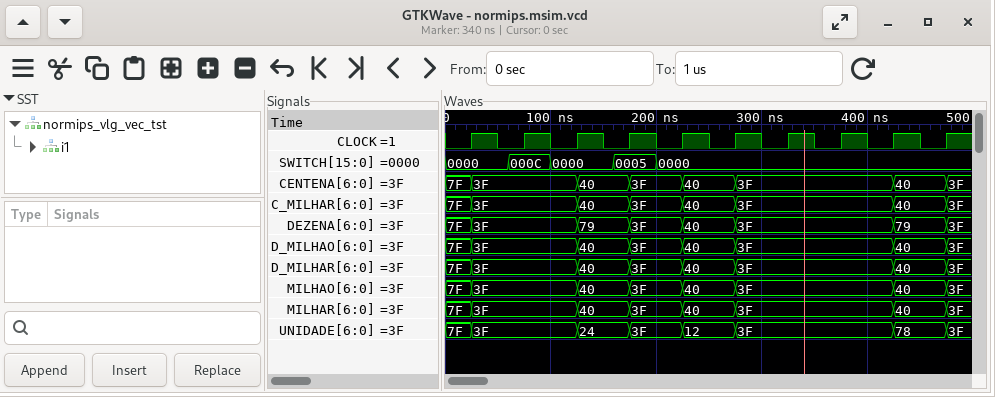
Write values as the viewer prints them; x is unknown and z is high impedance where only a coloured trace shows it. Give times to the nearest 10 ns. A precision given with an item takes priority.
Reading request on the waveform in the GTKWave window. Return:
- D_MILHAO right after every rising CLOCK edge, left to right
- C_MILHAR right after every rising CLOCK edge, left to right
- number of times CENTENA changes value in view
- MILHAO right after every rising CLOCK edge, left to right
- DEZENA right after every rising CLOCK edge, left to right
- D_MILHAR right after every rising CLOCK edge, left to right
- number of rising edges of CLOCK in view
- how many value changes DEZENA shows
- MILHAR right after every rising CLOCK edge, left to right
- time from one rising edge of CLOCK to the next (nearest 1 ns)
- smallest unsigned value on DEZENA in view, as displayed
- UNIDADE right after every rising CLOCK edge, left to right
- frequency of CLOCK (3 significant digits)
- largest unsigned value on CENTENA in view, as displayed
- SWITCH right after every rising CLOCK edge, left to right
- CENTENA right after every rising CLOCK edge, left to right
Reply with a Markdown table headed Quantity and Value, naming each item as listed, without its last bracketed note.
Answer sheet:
| Quantity | Value |
|---|---|
| D_MILHAO right after every rising CLOCK edge, left to right | 3F, 3F, 40, 3F, 40, 3F, 3F, 3F, 40, 3F |
| C_MILHAR right after every rising CLOCK edge, left to right | 3F, 3F, 40, 3F, 40, 3F, 3F, 3F, 40, 3F |
| number of times CENTENA changes value in view | 7 |
| MILHAO right after every rising CLOCK edge, left to right | 3F, 3F, 40, 3F, 40, 3F, 3F, 3F, 40, 3F |
| DEZENA right after every rising CLOCK edge, left to right | 3F, 3F, 79, 3F, 40, 3F, 3F, 3F, 79, 3F |
| D_MILHAR right after every rising CLOCK edge, left to right | 3F, 3F, 40, 3F, 40, 3F, 3F, 3F, 40, 3F |
| number of rising edges of CLOCK in view | 10 |
| how many value changes DEZENA shows | 7 |
| MILHAR right after every rising CLOCK edge, left to right | 3F, 3F, 40, 3F, 40, 3F, 3F, 3F, 40, 3F |
| time from one rising edge of CLOCK to the next | 50 ns |
| smallest unsigned value on DEZENA in view, as displayed | 3F |
| UNIDADE right after every rising CLOCK edge, left to right | 3F, 3F, 24, 3F, 12, 3F, 3F, 3F, 78, 3F |
| frequency of CLOCK | 20.0 MHz |
| largest unsigned value on CENTENA in view, as displayed | 7F |
| SWITCH right after every rising CLOCK edge, left to right | 0000, 000C, 0000, 0005, 0000, 0000, 0000, 0000, 0000, 0000 |
| CENTENA right after every rising CLOCK edge, left to right | 3F, 3F, 40, 3F, 40, 3F, 3F, 3F, 40, 3F |
